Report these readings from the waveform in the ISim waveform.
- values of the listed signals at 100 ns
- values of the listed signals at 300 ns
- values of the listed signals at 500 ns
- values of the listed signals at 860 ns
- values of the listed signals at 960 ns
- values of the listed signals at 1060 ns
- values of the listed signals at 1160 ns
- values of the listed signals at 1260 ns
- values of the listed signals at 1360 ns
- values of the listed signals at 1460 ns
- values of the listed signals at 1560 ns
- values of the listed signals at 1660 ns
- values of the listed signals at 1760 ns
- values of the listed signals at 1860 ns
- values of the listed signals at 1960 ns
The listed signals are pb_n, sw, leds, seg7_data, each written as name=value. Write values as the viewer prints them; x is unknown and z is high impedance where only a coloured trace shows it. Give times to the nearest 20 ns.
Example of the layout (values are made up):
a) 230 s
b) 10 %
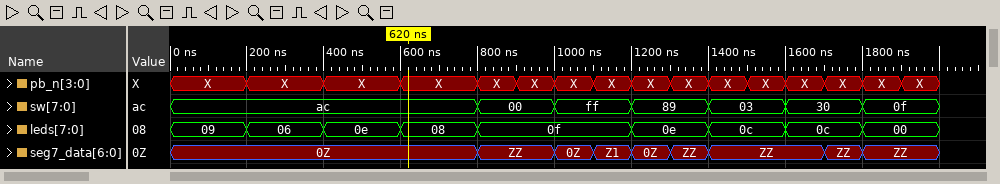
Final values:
a) pb_n=X, sw=ac, leds=09, seg7_data=0Z
b) pb_n=X, sw=ac, leds=06, seg7_data=0Z
c) pb_n=X, sw=ac, leds=0e, seg7_data=0Z
d) pb_n=X, sw=00, leds=0f, seg7_data=ZZ
e) pb_n=X, sw=00, leds=0f, seg7_data=ZZ
f) pb_n=X, sw=ff, leds=0f, seg7_data=0Z
g) pb_n=X, sw=ff, leds=0f, seg7_data=Z1
h) pb_n=X, sw=89, leds=0e, seg7_data=0Z
i) pb_n=X, sw=89, leds=0e, seg7_data=ZZ
j) pb_n=X, sw=03, leds=0c, seg7_data=ZZ
k) pb_n=X, sw=03, leds=0c, seg7_data=ZZ
l) pb_n=X, sw=30, leds=0c, seg7_data=ZZ
m) pb_n=X, sw=30, leds=0c, seg7_data=ZZ
n) pb_n=X, sw=0f, leds=00, seg7_data=ZZ
o) pb_n=X, sw=0f, leds=00, seg7_data=ZZ
